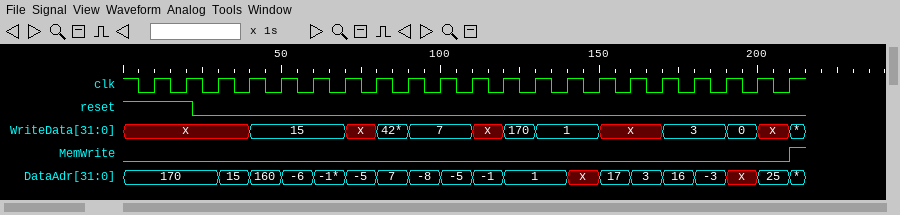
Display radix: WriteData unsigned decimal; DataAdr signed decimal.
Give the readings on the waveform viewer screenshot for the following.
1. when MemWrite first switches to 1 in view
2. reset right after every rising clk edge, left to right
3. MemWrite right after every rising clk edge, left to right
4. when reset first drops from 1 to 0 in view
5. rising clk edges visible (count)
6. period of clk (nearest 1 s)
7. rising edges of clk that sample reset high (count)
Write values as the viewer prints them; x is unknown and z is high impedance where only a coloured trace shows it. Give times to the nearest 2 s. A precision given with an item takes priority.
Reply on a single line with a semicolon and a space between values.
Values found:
210 s; 1 1 0 0 0 0 0 0 0 0 0 0 0 0 0 0 0 0 0 0 0; 0 0 0 0 0 0 0 0 0 0 0 0 0 0 0 0 0 0 0 0 1; 22 s; 21; 10 s; 2
